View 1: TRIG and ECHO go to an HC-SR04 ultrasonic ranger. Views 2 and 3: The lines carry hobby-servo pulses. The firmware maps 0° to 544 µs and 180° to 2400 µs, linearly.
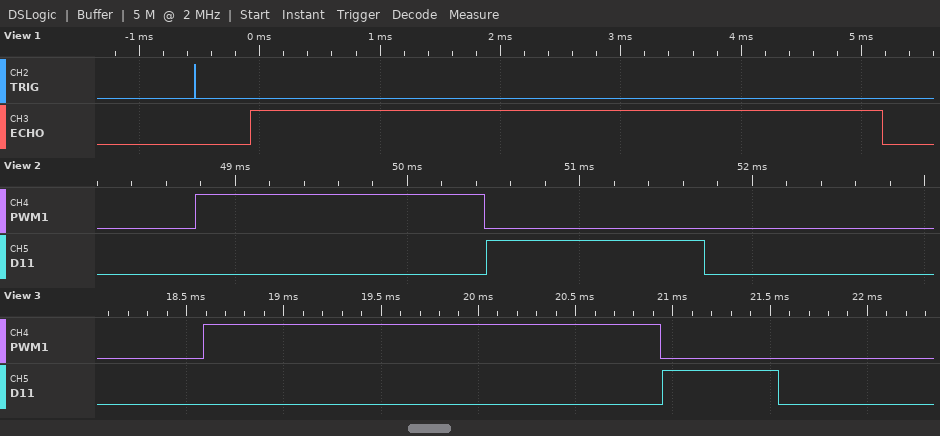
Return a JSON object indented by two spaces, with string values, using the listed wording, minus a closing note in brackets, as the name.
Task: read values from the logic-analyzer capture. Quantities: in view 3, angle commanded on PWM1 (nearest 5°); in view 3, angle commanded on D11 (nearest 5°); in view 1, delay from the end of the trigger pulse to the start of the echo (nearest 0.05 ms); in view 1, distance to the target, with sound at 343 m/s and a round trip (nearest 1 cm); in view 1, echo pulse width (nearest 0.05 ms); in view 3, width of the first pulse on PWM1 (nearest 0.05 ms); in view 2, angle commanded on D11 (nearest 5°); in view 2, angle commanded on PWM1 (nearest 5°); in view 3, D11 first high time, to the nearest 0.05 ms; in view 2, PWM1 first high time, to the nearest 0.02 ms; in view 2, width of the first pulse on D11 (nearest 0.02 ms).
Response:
{
  "in view 3, angle commanded on PWM1": "175°",
  "in view 3, angle commanded on D11": "5°",
  "in view 1, delay from the end of the trigger pulse to the start of the echo": "0.45 ms",
  "in view 1, distance to the target, with sound at 343 m/s and a round trip": "90 cm",
  "in view 1, echo pulse width": "5.25 ms",
  "in view 3, width of the first pulse on PWM1": "2.35 ms",
  "in view 2, angle commanded on D11": "70°",
  "in view 2, angle commanded on PWM1": "110°",
  "in view 3, D11 first high time, to the nearest 0.05 ms": "0.60 ms",
  "in view 2, PWM1 first high time, to the nearest 0.02 ms": "1.68 ms",
  "in view 2, width of the first pulse on D11": "1.26 ms"
}
